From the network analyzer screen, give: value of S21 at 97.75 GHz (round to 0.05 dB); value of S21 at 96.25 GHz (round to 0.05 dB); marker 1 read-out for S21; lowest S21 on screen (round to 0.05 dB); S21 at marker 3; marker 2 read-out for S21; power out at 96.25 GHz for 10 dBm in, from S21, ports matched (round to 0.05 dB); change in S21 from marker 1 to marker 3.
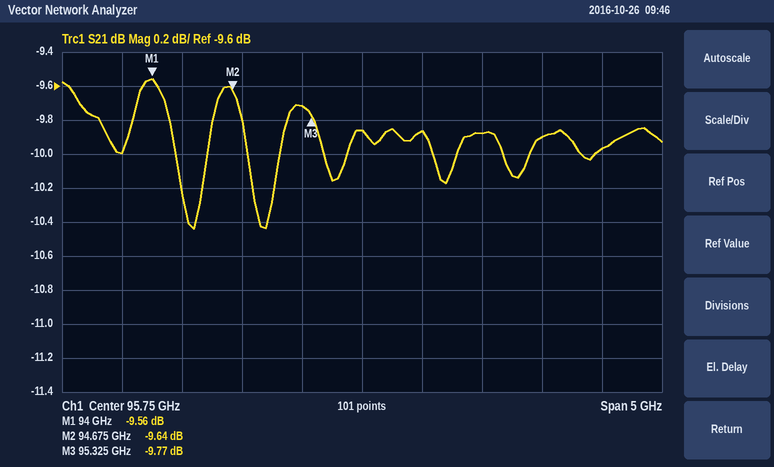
-9.95 dB
-9.85 dB
-9.56 dB
-10.45 dB
-9.77 dB
-9.64 dB
0.15 dBm
-0.21 dB
